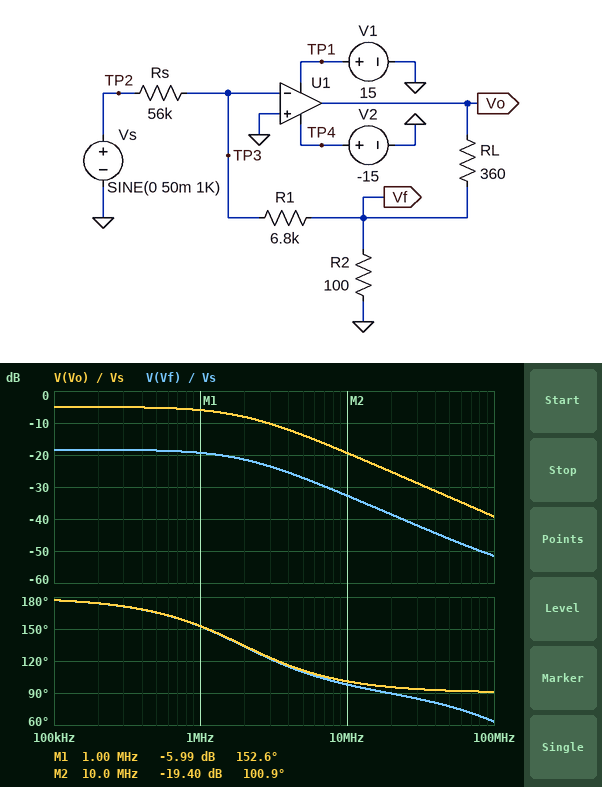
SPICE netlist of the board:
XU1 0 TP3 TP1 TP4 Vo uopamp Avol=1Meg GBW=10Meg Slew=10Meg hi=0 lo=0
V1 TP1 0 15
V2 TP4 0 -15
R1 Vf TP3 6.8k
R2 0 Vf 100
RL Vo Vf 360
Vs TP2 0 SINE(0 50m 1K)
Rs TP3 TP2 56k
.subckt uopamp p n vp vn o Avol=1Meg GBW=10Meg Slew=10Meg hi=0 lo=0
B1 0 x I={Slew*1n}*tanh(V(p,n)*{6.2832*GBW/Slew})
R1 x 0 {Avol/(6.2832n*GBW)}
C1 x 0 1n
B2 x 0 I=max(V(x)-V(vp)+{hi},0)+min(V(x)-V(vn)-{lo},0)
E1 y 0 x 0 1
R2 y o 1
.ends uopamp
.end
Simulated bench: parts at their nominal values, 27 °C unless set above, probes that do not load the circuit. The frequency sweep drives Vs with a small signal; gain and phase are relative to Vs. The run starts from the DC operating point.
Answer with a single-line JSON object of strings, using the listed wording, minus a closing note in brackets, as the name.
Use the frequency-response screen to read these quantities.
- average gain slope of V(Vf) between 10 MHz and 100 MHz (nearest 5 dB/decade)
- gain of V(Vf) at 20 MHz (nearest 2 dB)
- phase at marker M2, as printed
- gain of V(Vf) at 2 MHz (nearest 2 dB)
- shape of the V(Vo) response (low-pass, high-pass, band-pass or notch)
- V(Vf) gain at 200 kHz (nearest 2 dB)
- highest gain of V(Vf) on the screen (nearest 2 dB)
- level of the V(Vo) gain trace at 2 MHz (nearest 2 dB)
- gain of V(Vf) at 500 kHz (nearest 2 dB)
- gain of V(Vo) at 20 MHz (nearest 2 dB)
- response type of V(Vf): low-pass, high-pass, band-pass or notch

{"average gain slope of V(Vf) between 10 MHz and 100 MHz": "-20 dB/decade", "gain of V(Vf) at 20 MHz": "-38 dB", "phase at marker M2, as printed": "100.9 deg", "gain of V(Vf) at 2 MHz": "-22 dB", "shape of the V(Vo) response": "low-pass", "V(Vf) gain at 200 kHz": "-18 dB", "highest gain of V(Vf) on the screen": "-18 dB", "level of the V(Vo) gain trace at 2 MHz": "-8 dB", "gain of V(Vf) at 500 kHz": "-18 dB", "gain of V(Vo) at 20 MHz": "-26 dB", "response type of V(Vf): low-pass, high-pass, band-pass or notch": "low-pass"}
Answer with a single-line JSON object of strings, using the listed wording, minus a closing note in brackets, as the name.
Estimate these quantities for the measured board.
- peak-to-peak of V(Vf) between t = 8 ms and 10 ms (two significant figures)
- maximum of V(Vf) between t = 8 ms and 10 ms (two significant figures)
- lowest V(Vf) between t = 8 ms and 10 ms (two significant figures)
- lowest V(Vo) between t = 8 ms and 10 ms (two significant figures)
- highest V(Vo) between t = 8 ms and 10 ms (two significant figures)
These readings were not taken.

{"peak-to-peak of V(Vf) between t = 8 ms and 10 ms": "12 mV", "maximum of V(Vf) between t = 8 ms and 10 ms": "6.1 mV", "lowest V(Vf) between t = 8 ms and 10 ms": "-6.1 mV", "lowest V(Vo) between t = 8 ms and 10 ms": "-28 mV", "highest V(Vo) between t = 8 ms and 10 ms": "28 mV"}
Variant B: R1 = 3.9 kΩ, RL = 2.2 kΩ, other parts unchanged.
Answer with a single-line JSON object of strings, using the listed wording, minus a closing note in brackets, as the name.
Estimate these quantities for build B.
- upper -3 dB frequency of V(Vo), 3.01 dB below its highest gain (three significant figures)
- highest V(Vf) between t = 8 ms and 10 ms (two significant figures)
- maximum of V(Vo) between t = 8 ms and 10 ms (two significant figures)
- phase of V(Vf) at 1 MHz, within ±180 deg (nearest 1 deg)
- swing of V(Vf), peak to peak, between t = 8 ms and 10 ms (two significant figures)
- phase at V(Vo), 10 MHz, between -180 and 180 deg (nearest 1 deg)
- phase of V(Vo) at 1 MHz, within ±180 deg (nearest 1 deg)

{"upper -3 dB frequency of V(Vo), 3.01 dB below its highest gain": "406 kHz", "highest V(Vf) between t = 8 ms and 10 ms": "3.5 mV", "maximum of V(Vo) between t = 8 ms and 10 ms": "82 mV", "phase of V(Vf) at 1 MHz, within ±180 deg": "109 deg", "swing of V(Vf), peak to peak, between t = 8 ms and 10 ms": "7.0 mV", "phase at V(Vo), 10 MHz, between -180 and 180 deg": "92 deg", "phase of V(Vo) at 1 MHz, within ±180 deg": "112 deg"}
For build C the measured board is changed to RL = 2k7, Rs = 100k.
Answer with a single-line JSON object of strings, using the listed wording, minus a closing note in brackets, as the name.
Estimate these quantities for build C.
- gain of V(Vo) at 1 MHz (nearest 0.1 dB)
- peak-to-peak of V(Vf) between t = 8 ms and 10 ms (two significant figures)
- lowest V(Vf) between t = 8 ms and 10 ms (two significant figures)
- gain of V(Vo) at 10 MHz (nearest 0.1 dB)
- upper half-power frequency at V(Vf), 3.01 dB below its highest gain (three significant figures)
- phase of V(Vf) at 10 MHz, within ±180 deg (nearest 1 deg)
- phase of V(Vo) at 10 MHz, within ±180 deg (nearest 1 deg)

{"gain of V(Vo) at 1 MHz": "-4.3 dB", "peak-to-peak of V(Vf) between t = 8 ms and 10 ms": "6.8 mV", "lowest V(Vf) between t = 8 ms and 10 ms": "-3.4 mV", "gain of V(Vo) at 10 MHz": "-23.8 dB", "upper half-power frequency at V(Vf), 3.01 dB below its highest gain": "334 kHz", "phase of V(Vf) at 10 MHz, within ±180 deg": "70 deg", "phase of V(Vo) at 10 MHz, within ±180 deg": "92 deg"}
